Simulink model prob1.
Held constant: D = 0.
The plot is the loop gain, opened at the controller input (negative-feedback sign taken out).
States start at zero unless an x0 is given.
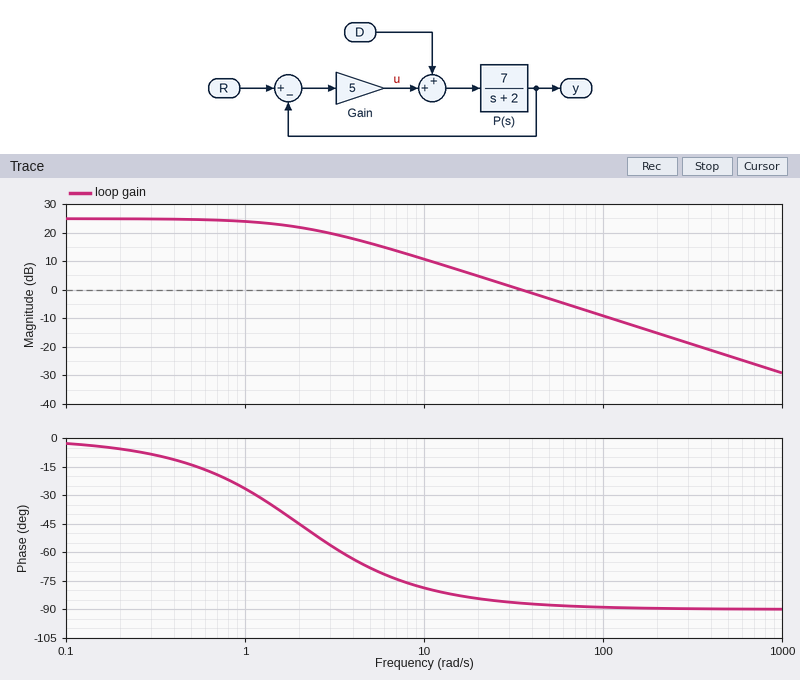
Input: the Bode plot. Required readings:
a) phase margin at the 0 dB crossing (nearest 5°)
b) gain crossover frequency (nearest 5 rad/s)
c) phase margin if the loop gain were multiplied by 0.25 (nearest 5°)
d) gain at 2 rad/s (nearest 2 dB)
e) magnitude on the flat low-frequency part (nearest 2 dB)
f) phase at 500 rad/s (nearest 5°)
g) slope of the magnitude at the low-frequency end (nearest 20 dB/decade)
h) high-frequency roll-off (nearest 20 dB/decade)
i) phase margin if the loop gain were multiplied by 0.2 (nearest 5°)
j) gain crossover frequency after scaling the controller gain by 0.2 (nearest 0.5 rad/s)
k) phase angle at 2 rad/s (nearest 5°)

95°
35 rad/s
105°
22 dB
24 dB
-90°
0 dB/decade
-20 dB/decade
105°
6.5 rad/s
-45°
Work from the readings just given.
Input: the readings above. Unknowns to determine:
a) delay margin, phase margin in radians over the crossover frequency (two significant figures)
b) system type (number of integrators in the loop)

0.047 s
0
